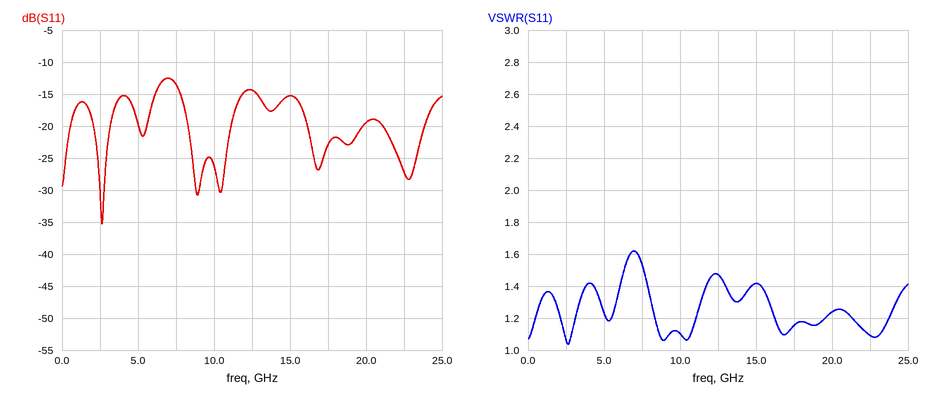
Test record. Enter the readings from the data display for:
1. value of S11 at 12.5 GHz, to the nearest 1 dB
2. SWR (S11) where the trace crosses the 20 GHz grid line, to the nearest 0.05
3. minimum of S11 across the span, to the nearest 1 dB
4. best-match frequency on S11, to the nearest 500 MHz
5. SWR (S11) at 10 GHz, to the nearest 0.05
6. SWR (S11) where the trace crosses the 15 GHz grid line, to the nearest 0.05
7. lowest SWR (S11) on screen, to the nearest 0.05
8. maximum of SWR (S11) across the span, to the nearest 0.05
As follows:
-14 dB
1.25
-35 dB
2.5 GHz
1.10
1.40
1.05
1.60
